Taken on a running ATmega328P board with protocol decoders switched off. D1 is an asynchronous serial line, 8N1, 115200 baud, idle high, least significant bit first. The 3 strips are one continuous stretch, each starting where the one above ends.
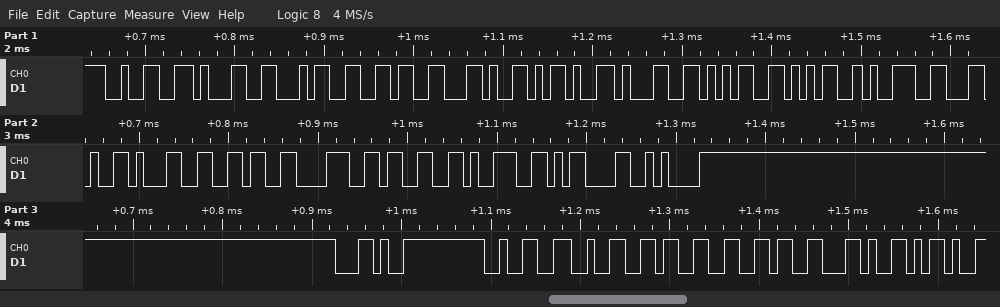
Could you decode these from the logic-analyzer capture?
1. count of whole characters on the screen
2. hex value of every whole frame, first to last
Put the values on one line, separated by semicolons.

25; 32 31 34 36 2C 2D 31 35 35 39 2C 31 36 38 33 39 0D 0A 2C 32 32 33 36 2C 2D
